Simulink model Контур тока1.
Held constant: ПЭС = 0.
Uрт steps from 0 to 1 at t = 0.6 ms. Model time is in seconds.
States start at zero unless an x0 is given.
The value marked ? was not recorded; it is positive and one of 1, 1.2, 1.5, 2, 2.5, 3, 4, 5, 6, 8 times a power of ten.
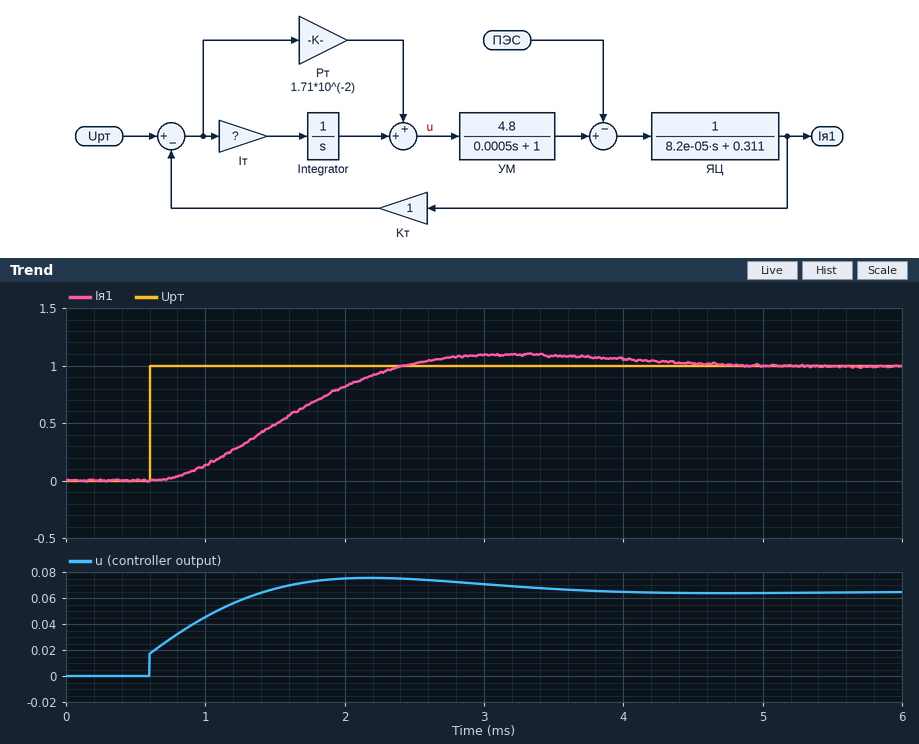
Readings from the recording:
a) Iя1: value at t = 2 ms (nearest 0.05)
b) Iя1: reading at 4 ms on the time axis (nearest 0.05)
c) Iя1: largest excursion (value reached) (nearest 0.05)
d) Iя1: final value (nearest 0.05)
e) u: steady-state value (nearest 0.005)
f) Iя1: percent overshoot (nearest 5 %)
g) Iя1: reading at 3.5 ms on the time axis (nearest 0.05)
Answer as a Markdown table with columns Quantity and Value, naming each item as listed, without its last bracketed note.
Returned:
| Quantity | Value |
|---|---|
| Iя1: value at t = 2 ms | 0.80 |
| Iя1: reading at 4 ms on the time axis | 1.05 |
| Iя1: largest excursion (value reached) | 1.10 |
| Iя1: final value | 1.00 |
| u: steady-state value | 0.065 |
| Iя1: percent overshoot | 10 % |
| Iя1: reading at 3.5 ms on the time axis | 1.10 |
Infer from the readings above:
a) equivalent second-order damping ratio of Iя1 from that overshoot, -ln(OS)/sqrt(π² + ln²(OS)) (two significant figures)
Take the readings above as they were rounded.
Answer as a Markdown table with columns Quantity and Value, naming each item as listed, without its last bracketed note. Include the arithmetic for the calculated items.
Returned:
| Quantity | Value |
|---|---|
| equivalent second-order damping ratio of Iя1 from that overshoot, -ln(OS)/sqrt(π² + ln²(OS)) | ln(0.1) = -2.303; 2.303 / sqrt(9.870 + 5.302) = 0.59 |
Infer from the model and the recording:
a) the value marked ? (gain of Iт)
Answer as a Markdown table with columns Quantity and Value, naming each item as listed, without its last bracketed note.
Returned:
| Quantity | Value |
|---|---|
| the value marked ? | 80 |
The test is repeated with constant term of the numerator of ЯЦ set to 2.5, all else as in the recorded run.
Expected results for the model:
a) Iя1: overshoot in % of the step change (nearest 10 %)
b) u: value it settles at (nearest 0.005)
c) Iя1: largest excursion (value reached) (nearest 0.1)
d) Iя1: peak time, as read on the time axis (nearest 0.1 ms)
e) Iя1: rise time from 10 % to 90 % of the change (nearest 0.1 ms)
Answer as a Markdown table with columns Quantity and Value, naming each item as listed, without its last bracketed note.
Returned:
| Quantity | Value |
|---|---|
| Iя1: overshoot in % of the step change | 30 % |
| u: value it settles at | 0.025 |
| Iя1: largest excursion (value reached) | 1.3 |
| Iя1: peak time, as read on the time axis | 2.0 ms |
| Iя1: rise time from 10 % to 90 % of the change | 0.6 ms |
